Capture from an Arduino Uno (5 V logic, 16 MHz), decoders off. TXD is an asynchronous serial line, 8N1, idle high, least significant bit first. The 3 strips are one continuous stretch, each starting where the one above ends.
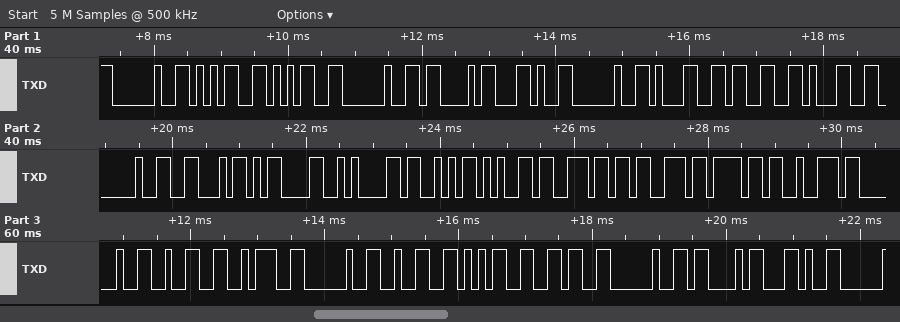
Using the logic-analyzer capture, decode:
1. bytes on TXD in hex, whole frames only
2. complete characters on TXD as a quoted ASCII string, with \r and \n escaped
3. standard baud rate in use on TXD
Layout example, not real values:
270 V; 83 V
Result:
20 35 35 20 43 2C 20 31 33 31 20 46 0D 0A 53 65 6E 73 6F 72 20 32 3A 20 32 35 36 20 43 2C; " 55 C, 131 F\r\nSensor 2: 256 C,"; 9600 baud
